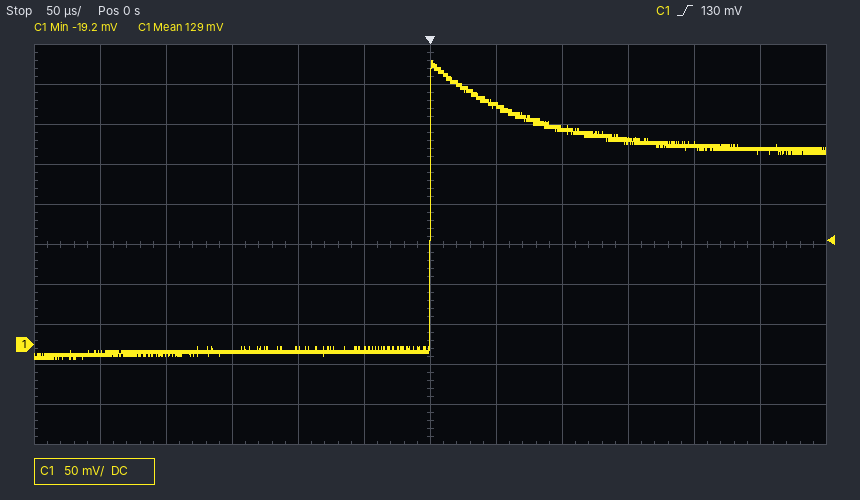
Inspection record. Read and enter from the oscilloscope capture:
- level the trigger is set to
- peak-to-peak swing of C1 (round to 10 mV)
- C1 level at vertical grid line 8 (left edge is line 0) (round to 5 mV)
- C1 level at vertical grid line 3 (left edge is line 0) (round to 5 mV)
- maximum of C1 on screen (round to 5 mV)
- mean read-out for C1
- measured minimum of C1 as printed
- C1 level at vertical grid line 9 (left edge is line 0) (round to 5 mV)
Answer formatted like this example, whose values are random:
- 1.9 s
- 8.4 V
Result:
- 130 mV
- 370 mV
- 270 mV
- -10 mV
- 355 mV
- 129 mV
- -19.2 mV
- 255 mV
